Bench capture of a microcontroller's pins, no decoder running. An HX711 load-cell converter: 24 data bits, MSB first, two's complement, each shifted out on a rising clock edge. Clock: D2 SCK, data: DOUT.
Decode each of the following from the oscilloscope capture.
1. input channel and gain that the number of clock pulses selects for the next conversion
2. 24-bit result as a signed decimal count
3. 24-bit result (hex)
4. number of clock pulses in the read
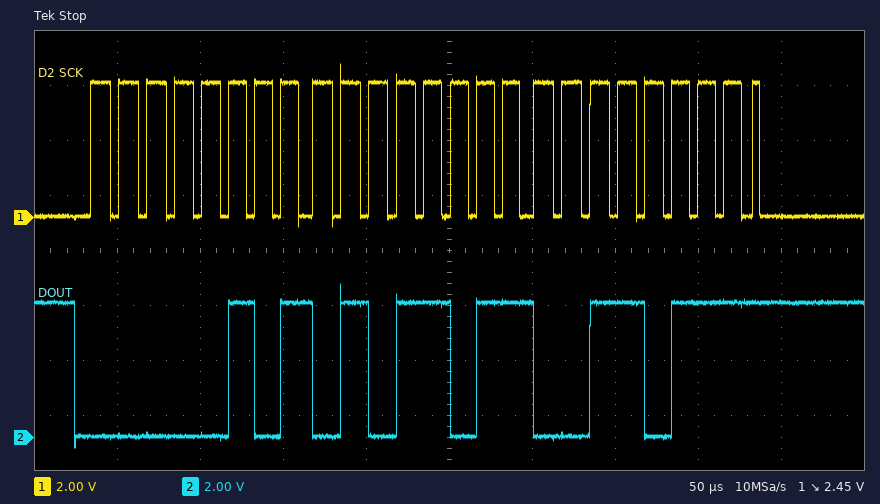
channel A, gain 128
351031
0x055B37
25
